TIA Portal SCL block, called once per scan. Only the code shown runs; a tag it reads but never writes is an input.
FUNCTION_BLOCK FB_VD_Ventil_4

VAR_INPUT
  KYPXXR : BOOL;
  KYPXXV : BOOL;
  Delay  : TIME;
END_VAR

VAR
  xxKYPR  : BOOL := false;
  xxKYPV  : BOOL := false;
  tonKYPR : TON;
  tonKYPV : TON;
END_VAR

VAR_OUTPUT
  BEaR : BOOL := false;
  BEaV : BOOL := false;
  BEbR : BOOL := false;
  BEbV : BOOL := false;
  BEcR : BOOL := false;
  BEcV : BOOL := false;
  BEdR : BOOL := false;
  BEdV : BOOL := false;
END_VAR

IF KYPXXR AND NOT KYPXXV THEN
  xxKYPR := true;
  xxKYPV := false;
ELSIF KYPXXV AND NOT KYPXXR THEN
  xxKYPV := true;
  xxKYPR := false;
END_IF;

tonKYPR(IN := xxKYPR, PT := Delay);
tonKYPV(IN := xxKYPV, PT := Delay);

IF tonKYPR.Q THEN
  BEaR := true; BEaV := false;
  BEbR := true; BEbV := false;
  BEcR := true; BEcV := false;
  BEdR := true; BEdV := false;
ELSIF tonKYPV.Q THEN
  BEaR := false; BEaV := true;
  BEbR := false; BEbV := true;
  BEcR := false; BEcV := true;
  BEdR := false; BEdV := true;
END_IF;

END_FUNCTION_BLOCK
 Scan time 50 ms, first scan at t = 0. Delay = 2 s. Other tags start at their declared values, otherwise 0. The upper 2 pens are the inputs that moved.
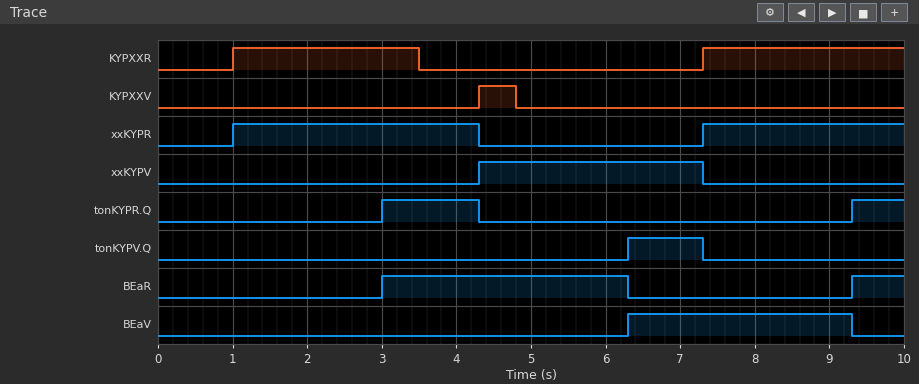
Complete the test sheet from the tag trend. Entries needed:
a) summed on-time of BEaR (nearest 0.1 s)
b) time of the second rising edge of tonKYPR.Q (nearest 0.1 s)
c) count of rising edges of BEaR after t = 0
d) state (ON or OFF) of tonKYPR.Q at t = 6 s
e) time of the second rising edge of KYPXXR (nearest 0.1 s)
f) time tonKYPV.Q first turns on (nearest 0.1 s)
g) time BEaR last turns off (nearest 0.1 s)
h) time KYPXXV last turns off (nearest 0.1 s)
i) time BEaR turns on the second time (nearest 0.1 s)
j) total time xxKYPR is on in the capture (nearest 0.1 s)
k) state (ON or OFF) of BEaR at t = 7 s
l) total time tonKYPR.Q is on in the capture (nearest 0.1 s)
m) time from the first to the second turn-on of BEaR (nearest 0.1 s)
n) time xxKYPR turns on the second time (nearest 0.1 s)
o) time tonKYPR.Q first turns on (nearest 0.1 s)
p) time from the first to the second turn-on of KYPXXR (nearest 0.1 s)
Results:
4.0 s
9.3 s
2
OFF
7.3 s
6.3 s
6.3 s
4.8 s
9.3 s
6.0 s
OFF
2.0 s
6.3 s
7.3 s
3.0 s
6.3 s
